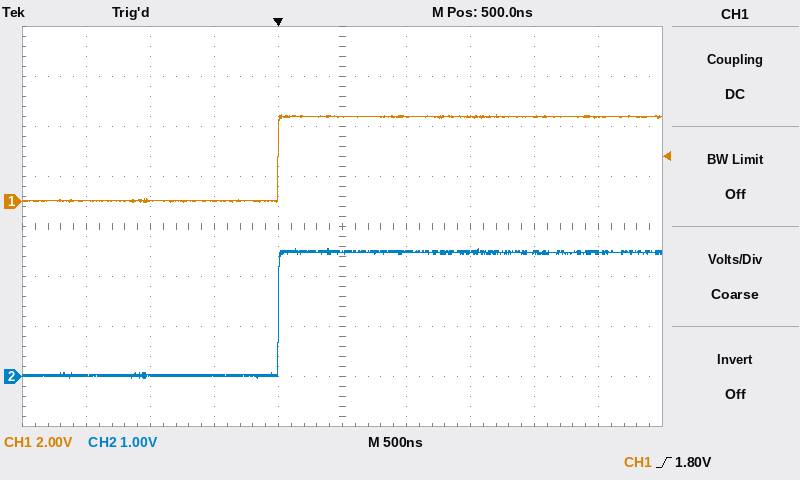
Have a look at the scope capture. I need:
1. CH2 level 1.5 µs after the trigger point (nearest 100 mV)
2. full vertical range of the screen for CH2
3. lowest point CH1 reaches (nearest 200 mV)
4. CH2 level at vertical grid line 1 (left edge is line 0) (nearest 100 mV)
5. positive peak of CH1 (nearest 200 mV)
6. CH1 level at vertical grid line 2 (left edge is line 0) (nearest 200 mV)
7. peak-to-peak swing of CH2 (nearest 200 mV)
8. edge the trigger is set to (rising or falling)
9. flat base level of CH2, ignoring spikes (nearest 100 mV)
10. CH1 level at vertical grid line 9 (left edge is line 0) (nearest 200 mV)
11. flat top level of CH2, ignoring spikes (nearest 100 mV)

2.5 V
8 V
0.0 V
0.0 V
3.4 V
0.0 V
2.6 V
rising
0.0 V
3.4 V
2.5 V
